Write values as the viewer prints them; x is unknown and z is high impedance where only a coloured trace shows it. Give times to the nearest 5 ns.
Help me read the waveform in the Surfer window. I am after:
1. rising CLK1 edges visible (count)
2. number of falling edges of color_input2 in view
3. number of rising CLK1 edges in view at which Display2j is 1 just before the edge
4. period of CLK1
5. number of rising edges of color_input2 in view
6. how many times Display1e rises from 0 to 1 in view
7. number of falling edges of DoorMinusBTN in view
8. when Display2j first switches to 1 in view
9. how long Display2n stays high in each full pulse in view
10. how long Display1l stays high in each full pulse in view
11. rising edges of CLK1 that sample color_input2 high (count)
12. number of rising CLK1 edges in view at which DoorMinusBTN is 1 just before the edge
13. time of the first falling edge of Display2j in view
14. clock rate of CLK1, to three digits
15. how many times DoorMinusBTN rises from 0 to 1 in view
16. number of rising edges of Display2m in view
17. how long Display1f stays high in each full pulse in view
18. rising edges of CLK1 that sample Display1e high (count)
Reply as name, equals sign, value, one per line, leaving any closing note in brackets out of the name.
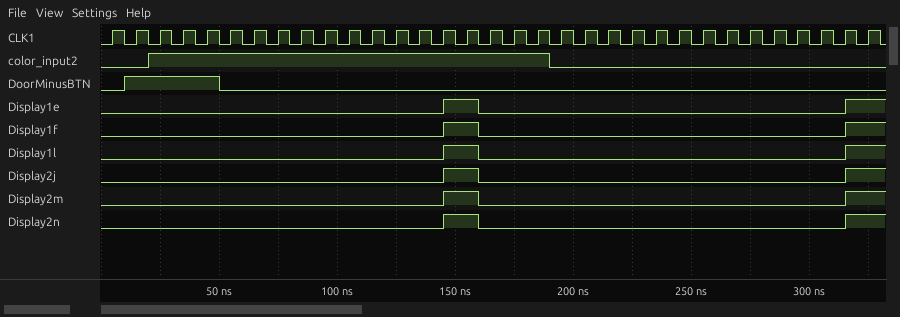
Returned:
rising CLK1 edges visible = 33
number of falling edges of color_input2 in view = 1
number of rising CLK1 edges in view at which Display2j is 1 just before the edge = 2
period of CLK1 = 10 ns
number of rising edges of color_input2 in view = 1
how many times Display1e rises from 0 to 1 in view = 2
number of falling edges of DoorMinusBTN in view = 1
when Display2j first switches to 1 in view = 145 ns
how long Display2n stays high in each full pulse in view = 15 ns
how long Display1l stays high in each full pulse in view = 15 ns
rising edges of CLK1 that sample color_input2 high = 17
number of rising CLK1 edges in view at which DoorMinusBTN is 1 just before the edge = 4
time of the first falling edge of Display2j in view = 160 ns
clock rate of CLK1, to three digits = 100 MHz
how many times DoorMinusBTN rises from 0 to 1 in view = 1
number of rising edges of Display2m in view = 2
how long Display1f stays high in each full pulse in view = 15 ns
rising edges of CLK1 that sample Display1e high = 2
